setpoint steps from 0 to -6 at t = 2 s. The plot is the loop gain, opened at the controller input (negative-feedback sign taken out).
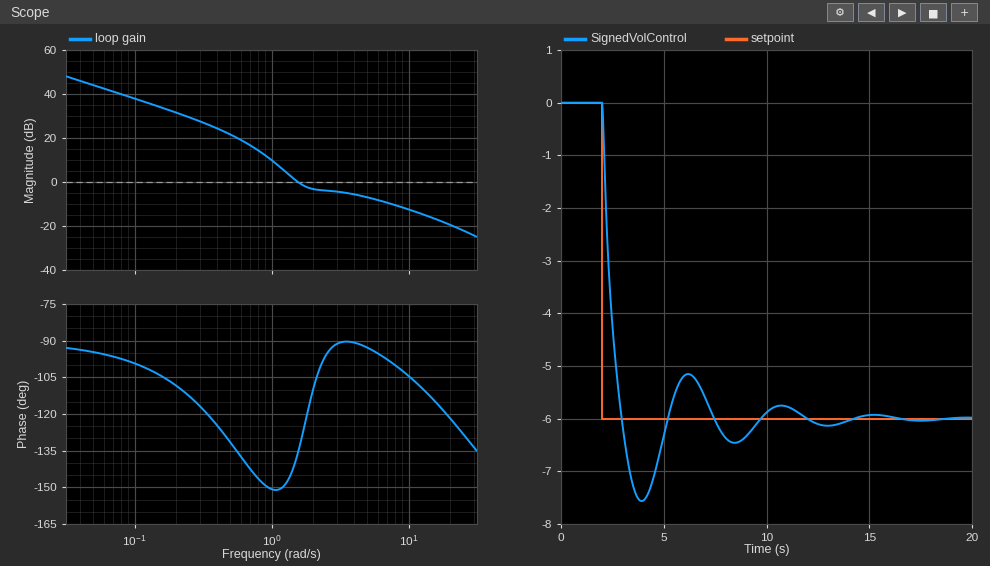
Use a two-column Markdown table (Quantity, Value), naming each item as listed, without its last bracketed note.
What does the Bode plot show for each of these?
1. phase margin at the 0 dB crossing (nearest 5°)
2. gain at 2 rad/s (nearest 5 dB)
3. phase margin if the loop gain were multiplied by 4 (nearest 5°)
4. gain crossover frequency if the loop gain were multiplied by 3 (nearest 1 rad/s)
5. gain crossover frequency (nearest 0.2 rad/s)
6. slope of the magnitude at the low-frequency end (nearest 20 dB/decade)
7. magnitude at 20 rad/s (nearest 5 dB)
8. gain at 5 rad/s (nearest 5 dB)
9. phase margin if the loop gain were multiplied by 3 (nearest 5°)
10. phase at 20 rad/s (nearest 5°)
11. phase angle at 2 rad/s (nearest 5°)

| Quantity | Value |
|---|---|
| phase margin at the 0 dB crossing | 45° |
| gain at 2 rad/s | -5 dB |
| phase margin if the loop gain were multiplied by 4 | 75° |
| gain crossover frequency if the loop gain were multiplied by 3 | 7 rad/s |
| gain crossover frequency | 1.6 rad/s |
| slope of the magnitude at the low-frequency end | -20 dB/decade |
| magnitude at 20 rad/s | -20 dB |
| gain at 5 rad/s | -5 dB |
| phase margin if the loop gain were multiplied by 3 | 80° |
| phase at 20 rad/s | -120° |
| phase angle at 2 rad/s | -110° |
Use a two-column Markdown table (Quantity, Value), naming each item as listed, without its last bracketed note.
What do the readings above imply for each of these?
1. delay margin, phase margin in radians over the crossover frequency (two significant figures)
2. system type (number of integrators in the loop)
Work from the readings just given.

| Quantity | Value |
|---|---|
| delay margin, phase margin in radians over the crossover frequency | 0.49 s |
| system type | 1 |
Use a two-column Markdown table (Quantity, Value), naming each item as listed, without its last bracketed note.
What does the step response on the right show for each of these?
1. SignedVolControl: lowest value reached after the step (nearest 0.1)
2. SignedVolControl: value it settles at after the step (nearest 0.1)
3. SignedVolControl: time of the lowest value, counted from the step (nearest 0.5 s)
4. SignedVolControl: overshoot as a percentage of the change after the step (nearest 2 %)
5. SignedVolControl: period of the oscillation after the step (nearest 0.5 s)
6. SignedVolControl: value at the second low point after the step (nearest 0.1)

| Quantity | Value |
|---|---|
| SignedVolControl: lowest value reached after the step | -7.6 |
| SignedVolControl: value it settles at after the step | -6.0 |
| SignedVolControl: time of the lowest value, counted from the step | 2.0 s |
| SignedVolControl: overshoot as a percentage of the change after the step | 26 % |
| SignedVolControl: period of the oscillation after the step | 4.5 s |
| SignedVolControl: value at the second low point after the step | -6.5 |
